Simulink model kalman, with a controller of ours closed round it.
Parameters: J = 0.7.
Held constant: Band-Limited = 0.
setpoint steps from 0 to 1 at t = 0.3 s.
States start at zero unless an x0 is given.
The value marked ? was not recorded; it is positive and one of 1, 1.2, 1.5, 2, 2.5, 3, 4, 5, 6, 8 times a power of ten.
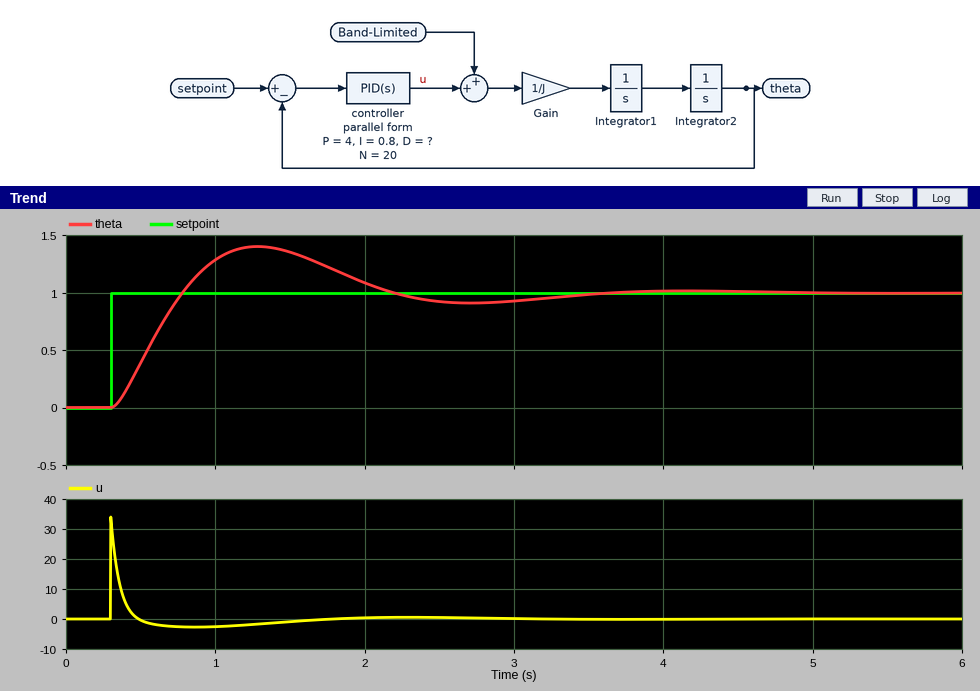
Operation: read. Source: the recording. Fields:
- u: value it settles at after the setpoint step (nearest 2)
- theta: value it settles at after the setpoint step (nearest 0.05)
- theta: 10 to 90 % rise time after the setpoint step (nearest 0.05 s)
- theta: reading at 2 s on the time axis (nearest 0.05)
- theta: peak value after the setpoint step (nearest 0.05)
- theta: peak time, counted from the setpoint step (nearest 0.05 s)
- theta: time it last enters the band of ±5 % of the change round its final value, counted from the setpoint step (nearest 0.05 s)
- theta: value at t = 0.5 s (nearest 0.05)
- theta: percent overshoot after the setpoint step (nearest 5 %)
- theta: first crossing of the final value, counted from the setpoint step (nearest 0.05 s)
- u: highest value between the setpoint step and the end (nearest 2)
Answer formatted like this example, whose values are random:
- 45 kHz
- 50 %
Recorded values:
- 0
- 1.00
- 0.35 s
- 1.10
- 1.40
- 1.00 s
- 2.90 s
- 0.40
- 40 %
- 0.50 s
- 34
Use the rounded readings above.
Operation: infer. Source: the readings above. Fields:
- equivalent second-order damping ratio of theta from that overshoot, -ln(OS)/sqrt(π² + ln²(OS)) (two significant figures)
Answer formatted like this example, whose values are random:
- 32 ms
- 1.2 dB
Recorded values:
- 0.28
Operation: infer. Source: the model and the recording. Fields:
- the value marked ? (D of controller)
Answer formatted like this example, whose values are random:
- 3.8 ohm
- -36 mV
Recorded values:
- 1.5
